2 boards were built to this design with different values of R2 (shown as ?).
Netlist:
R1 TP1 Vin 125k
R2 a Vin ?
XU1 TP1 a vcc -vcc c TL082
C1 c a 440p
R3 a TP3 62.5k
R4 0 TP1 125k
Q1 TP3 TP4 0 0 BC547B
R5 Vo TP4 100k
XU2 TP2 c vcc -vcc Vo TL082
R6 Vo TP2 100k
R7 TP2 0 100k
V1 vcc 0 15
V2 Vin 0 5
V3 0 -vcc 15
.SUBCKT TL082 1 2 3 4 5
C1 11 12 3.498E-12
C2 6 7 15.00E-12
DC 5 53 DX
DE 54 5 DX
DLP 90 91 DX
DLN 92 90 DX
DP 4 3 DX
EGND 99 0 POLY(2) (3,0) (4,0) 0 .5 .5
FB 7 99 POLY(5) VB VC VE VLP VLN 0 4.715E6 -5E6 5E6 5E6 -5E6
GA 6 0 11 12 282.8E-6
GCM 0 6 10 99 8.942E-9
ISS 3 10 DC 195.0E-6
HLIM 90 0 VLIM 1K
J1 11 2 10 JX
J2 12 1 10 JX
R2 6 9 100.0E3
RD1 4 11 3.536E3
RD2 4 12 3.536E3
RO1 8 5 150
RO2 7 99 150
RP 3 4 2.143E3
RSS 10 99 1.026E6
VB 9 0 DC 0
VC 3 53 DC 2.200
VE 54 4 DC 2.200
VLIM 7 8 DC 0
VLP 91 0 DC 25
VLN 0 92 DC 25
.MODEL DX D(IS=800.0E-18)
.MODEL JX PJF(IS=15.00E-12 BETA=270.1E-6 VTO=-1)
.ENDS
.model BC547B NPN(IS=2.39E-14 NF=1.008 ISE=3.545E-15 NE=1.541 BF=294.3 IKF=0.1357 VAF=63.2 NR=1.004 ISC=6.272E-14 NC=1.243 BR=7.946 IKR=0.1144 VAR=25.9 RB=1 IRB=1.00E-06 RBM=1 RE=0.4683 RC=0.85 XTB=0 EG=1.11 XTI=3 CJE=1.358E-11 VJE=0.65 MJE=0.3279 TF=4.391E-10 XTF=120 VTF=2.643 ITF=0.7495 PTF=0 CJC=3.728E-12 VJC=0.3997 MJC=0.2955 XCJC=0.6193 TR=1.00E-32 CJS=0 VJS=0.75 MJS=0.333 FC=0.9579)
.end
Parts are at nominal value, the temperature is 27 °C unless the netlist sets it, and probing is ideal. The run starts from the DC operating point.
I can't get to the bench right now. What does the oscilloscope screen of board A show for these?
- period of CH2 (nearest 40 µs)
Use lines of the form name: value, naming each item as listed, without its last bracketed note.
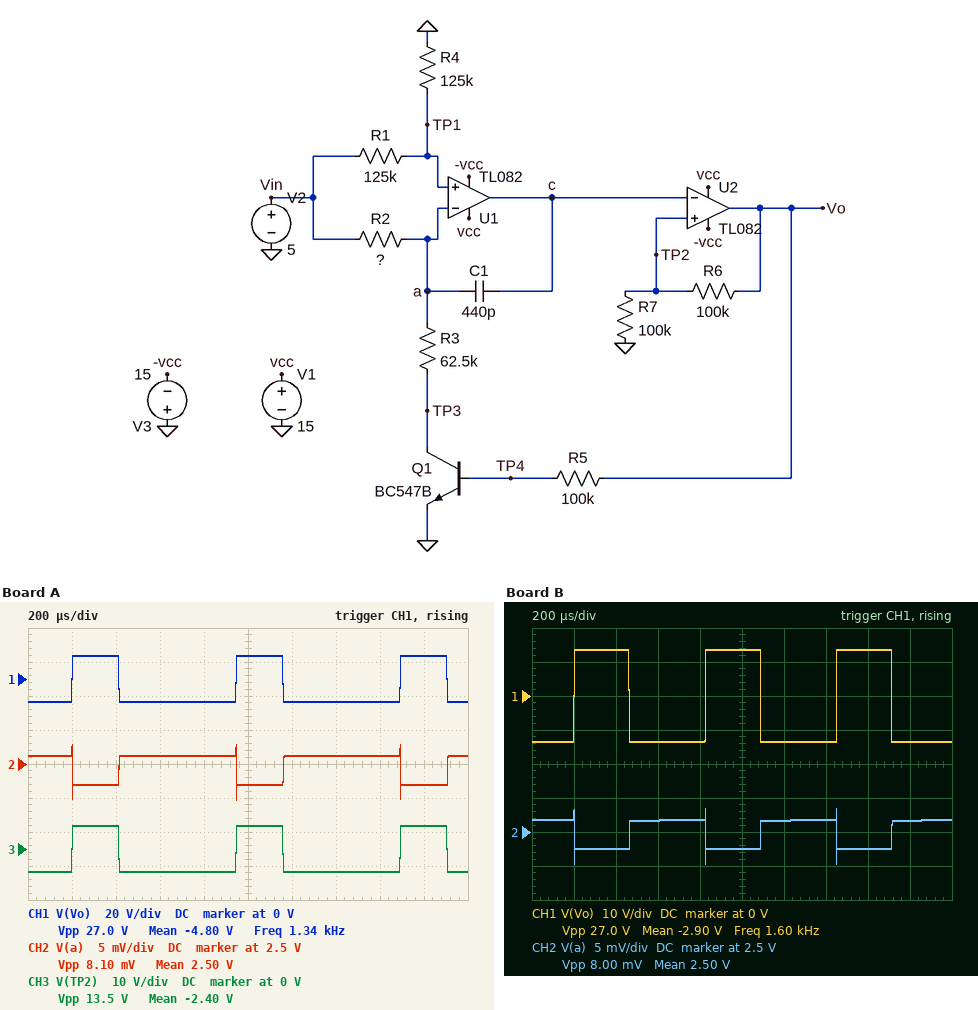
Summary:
period of CH2: 760 µs
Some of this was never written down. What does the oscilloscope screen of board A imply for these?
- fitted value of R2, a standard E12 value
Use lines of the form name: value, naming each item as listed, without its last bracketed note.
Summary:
fitted value of R2, a standard E12 value: 220 kΩ
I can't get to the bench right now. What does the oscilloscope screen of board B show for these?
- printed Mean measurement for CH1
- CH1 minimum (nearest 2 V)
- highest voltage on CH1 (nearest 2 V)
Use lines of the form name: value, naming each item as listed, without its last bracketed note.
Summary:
printed Mean measurement for CH1: -2.90 V
CH1 minimum: -14 V
highest voltage on CH1: 14 V
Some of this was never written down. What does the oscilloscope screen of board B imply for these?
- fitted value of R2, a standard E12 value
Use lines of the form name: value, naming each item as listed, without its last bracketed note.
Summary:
fitted value of R2, a standard E12 value: 150 kΩ
